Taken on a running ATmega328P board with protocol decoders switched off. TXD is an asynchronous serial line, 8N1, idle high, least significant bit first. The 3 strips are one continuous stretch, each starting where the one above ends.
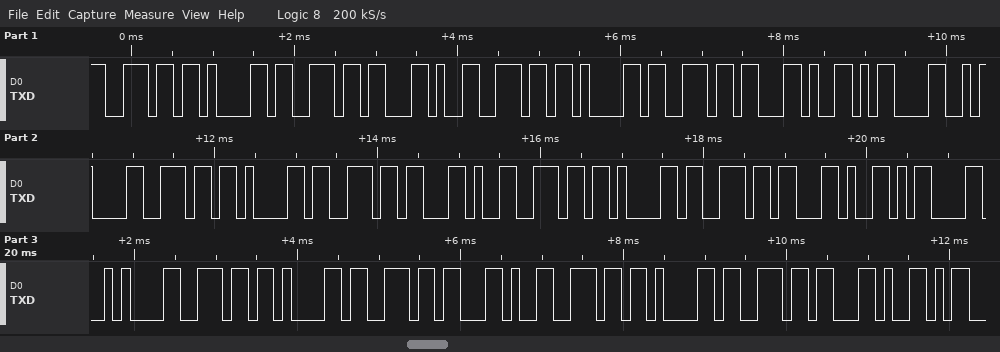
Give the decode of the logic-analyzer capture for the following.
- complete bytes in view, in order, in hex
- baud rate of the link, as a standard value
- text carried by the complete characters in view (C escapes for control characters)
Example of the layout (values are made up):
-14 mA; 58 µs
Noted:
6E 61 6E 2C 6E 61 6E 2C 0D 0A 6E 61 6E 2C 6E 61 6E 2C 0D 0A 6E 61 6E 2C 6E 61 6E 2C; 9600 baud; "nan,nan,\r\nnan,nan,\r\nnan,nan,"
